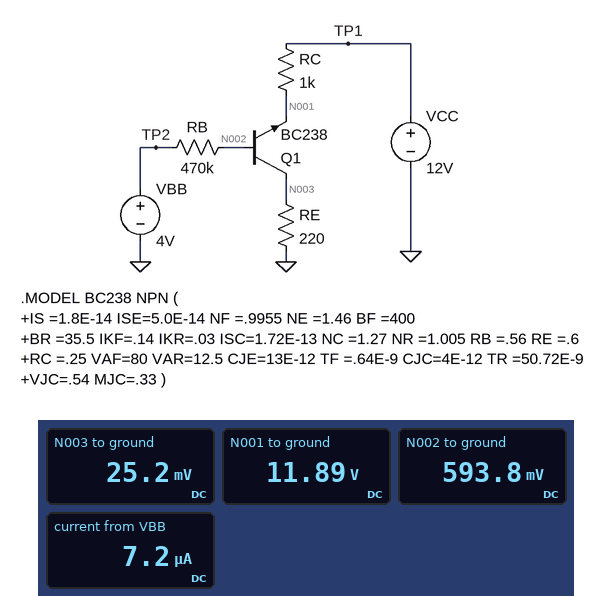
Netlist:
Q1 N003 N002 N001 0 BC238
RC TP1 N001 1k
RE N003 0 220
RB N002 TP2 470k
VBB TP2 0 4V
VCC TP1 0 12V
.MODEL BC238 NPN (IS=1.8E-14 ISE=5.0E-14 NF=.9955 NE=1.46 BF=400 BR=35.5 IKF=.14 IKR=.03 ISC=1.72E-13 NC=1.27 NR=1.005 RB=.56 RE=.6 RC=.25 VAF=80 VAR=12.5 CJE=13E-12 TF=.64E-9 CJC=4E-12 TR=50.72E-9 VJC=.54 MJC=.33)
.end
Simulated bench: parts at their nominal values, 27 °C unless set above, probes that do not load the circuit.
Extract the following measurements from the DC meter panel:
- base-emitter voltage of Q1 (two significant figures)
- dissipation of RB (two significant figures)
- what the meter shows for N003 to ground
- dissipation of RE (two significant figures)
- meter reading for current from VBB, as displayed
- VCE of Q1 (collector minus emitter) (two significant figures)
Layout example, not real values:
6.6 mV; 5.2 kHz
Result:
-11 V; 25 µW; 25.2 mV; 2.9 µW; 7.2 µA; -12 V
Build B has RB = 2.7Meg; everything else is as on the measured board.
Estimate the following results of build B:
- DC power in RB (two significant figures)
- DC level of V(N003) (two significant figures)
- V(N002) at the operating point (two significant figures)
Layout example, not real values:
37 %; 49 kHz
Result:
4.5 µW; 3.3 mV; 520 mV
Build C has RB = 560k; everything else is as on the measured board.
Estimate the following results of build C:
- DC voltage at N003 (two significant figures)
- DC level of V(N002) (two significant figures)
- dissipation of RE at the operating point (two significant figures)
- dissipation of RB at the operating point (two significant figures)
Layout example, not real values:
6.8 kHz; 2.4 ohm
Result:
21 mV; 580 mV; 1.9 µW; 21 µW
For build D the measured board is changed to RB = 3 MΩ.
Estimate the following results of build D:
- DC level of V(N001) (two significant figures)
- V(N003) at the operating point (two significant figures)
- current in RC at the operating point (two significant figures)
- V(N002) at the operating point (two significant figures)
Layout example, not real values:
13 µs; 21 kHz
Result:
12 V; 2.9 mV; 12 µA; 510 mV
